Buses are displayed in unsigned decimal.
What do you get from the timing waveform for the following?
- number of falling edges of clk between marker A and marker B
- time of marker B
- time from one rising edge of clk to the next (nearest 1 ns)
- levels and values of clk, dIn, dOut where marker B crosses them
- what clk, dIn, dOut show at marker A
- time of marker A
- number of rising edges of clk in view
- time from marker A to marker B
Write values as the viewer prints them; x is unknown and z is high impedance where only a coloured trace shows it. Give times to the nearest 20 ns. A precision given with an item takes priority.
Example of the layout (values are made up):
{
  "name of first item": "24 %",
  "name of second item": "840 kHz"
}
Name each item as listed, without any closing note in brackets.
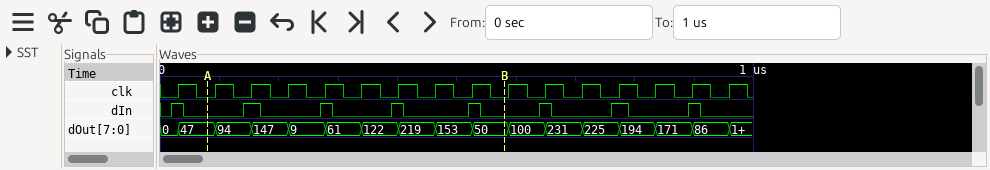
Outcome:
{
  "number of falling edges of clk between marker A and marker B": "8",
  "time of marker B": "580 ns",
  "time from one rising edge of clk to the next": "62 ns",
  "levels and values of clk, dIn, dOut where marker B crosses them": "clk=0, dIn=0, dOut=50",
  "what clk, dIn, dOut show at marker A": "clk=0, dIn=0, dOut=47",
  "time of marker A": "80 ns",
  "number of rising edges of clk in view": "16",
  "time from marker A to marker B": "500 ns"
}
